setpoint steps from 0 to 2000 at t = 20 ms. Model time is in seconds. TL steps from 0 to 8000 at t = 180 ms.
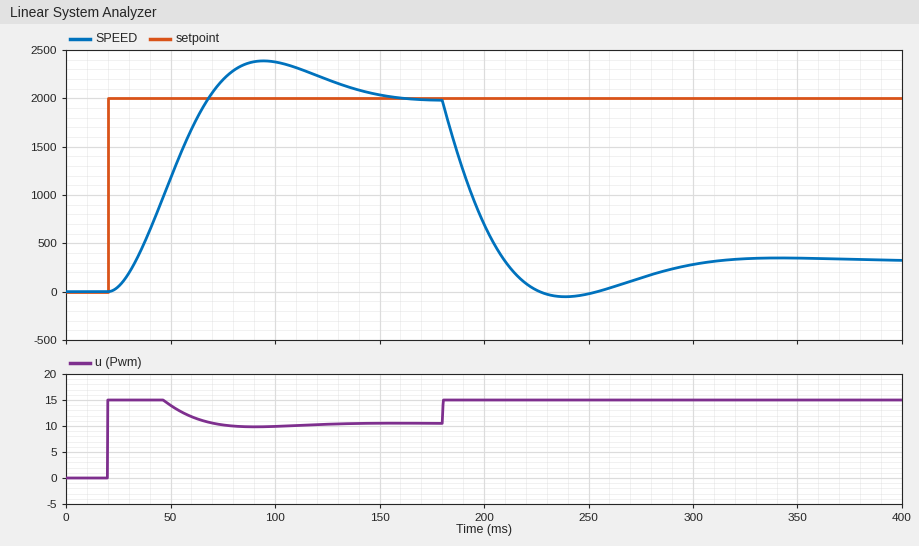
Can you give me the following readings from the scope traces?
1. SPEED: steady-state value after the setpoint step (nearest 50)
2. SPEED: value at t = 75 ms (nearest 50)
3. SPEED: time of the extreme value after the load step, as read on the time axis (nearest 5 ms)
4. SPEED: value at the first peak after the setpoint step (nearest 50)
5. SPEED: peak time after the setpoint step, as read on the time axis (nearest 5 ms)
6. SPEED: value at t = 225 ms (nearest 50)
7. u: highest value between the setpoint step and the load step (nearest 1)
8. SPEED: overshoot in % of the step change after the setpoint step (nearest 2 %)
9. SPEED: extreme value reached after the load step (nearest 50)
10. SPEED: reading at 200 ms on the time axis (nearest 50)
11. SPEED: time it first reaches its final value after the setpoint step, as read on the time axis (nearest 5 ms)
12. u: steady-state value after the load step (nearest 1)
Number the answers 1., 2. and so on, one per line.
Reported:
1. 2000
2. 2200
3. 240 ms
4. 2400
5. 95 ms
6. 0
7. 15
8. 20 %
9. -50
10. 700
11. 70 ms
12. 15
